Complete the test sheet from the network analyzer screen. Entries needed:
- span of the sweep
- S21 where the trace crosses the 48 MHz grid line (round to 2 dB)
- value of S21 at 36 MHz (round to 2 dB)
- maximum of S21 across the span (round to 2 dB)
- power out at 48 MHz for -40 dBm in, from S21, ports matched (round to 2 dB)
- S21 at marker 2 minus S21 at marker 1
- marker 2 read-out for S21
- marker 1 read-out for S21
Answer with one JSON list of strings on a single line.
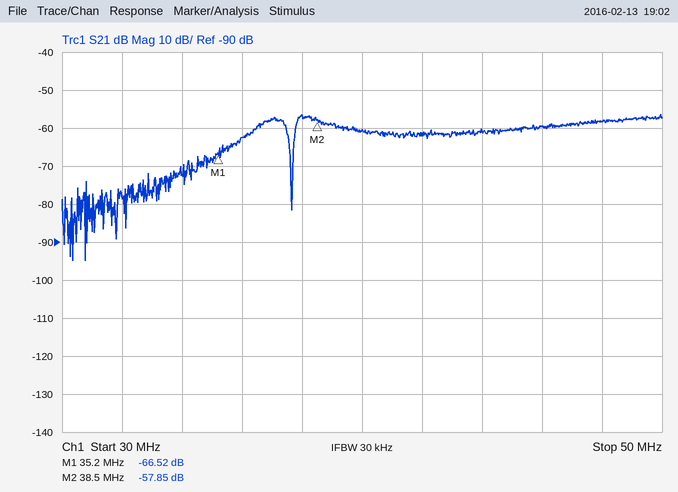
["20 MHz", "-58 dB", "-62 dB", "-56 dB", "-98 dBm", "8.67 dB", "-57.85 dB", "-66.52 dB"]
